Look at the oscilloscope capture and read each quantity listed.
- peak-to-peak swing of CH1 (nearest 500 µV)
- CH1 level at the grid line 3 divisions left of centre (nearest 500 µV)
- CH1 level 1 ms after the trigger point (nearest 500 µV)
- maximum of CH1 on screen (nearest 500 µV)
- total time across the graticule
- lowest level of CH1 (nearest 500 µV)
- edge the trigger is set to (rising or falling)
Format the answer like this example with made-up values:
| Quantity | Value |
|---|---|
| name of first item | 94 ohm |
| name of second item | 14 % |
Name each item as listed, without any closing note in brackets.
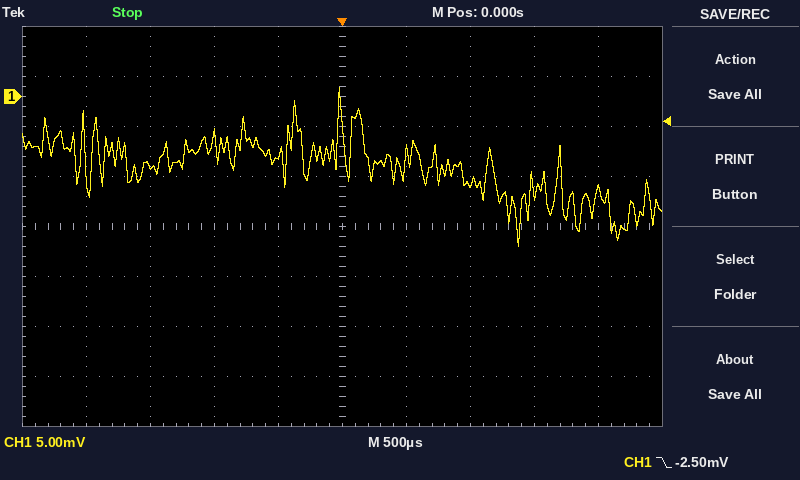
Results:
| Quantity | Value |
|---|---|
| peak-to-peak swing of CH1 | 16.0 mV |
| CH1 level at the grid line 3 divisions left of centre | -7.0 mV |
| CH1 level 1 ms after the trigger point | -8.5 mV |
| maximum of CH1 on screen | 1.0 mV |
| total time across the graticule | 5 ms |
| lowest level of CH1 | -15.0 mV |
| edge the trigger is set to | falling |
